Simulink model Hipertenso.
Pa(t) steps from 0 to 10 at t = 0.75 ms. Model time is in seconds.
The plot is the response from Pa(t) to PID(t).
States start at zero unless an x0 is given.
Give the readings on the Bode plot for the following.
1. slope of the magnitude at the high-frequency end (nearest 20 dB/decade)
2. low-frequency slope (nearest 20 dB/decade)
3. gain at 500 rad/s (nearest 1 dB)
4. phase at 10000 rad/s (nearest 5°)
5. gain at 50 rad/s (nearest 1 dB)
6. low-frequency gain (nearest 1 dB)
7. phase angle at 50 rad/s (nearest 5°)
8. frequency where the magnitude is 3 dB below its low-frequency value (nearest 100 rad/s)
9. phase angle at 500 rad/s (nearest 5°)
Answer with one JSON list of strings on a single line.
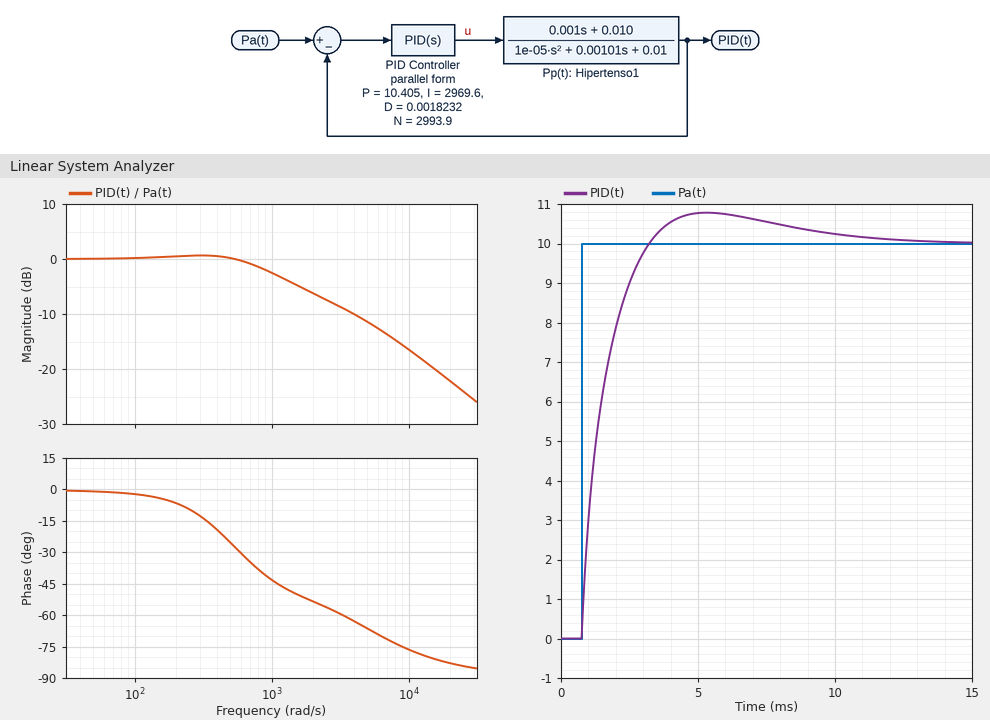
["-20 dB/decade", "0 dB/decade", "0 dB", "-75°", "0 dB", "0 dB", "0°", "1100 rad/s", "-25°"]
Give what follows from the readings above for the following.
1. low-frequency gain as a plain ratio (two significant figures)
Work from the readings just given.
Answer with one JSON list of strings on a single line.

["1.0"]
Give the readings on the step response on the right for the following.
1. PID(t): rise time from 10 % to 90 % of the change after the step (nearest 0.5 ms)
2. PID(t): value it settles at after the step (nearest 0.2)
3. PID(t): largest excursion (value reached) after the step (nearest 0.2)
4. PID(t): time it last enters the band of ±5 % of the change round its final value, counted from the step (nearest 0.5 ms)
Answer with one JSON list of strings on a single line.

["1.5 ms", "10.0", "10.8", "7.0 ms"]
